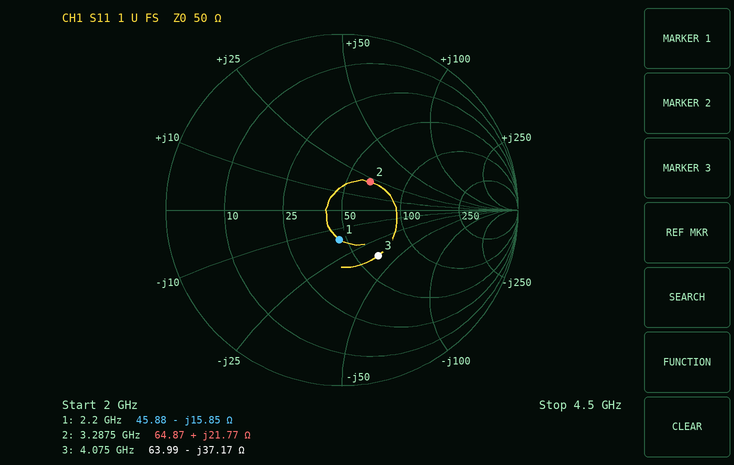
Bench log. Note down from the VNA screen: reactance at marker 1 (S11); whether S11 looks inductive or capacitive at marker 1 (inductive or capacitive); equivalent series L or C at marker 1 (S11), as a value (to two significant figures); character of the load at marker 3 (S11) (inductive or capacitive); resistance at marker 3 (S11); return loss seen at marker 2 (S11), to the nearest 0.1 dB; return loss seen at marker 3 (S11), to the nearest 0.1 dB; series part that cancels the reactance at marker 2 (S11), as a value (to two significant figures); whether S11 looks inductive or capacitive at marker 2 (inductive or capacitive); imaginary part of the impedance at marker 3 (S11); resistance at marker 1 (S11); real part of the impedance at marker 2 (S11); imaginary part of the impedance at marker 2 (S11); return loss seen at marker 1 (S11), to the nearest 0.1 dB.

-15.85 Ω
capacitive
4.6 pF
capacitive
63.99 Ω
12.9 dB
9.6 dB
2.2 pF
inductive
-37.17 Ω
45.88 Ω
64.87 Ω
+21.77 Ω
15.5 dB
